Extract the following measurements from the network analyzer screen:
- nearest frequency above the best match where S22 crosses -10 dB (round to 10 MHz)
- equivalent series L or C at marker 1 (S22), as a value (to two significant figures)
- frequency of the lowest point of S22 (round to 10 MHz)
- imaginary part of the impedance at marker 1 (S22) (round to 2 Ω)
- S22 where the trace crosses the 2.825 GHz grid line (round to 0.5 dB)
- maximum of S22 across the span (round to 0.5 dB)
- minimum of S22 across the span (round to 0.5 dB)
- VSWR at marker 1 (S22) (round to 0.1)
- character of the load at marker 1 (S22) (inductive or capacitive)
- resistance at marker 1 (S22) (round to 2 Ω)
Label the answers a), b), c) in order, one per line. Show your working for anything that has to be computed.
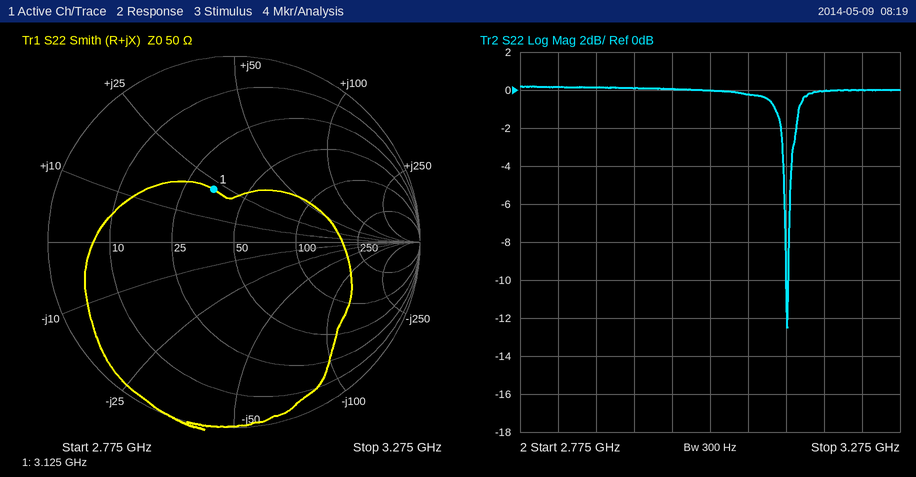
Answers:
a) 3.13 GHz
b) L = 22 Ω/(2π × 3.125 GHz) ≈ 1.1 nH
c) 3.13 GHz
d) +22 Ω
e) 0.0 dB
f) 0.0 dB
g) -12.5 dB
h) 1.9
i) inductive
j) 34 Ω
